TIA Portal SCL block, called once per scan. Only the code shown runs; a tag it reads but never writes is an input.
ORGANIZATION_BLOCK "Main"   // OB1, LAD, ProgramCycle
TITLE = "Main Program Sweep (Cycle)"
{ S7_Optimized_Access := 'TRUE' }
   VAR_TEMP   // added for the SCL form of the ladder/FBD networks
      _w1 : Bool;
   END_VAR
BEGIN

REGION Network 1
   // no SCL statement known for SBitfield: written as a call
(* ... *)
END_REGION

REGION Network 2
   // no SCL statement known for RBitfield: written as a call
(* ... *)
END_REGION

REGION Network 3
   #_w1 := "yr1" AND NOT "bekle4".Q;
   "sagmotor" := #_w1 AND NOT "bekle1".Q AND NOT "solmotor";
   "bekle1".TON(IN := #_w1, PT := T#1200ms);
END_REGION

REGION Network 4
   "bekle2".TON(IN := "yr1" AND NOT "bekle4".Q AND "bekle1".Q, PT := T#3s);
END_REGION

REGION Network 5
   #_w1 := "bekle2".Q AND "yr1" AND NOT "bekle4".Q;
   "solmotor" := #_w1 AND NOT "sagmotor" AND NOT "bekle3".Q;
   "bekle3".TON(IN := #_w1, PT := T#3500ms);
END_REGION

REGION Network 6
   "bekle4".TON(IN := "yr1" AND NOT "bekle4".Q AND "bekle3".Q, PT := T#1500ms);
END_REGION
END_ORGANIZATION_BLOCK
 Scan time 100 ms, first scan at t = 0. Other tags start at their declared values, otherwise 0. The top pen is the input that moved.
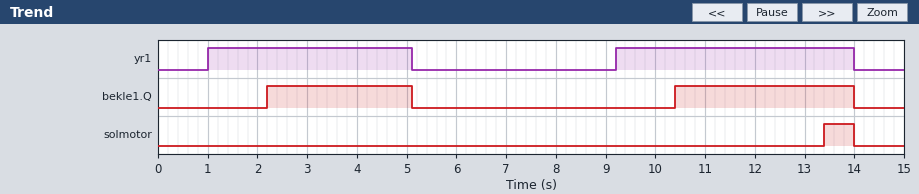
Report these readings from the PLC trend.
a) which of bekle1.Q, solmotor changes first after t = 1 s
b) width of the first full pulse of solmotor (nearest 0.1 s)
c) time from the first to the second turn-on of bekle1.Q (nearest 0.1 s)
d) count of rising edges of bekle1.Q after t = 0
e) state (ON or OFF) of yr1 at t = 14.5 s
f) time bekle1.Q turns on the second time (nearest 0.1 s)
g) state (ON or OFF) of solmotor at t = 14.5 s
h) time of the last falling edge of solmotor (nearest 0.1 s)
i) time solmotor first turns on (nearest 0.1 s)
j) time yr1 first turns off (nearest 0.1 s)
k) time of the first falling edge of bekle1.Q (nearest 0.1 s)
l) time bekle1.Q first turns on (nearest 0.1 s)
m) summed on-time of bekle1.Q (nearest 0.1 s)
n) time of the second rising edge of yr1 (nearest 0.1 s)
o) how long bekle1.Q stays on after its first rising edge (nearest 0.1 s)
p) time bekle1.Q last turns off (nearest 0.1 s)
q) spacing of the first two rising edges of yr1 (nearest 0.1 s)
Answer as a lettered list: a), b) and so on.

a) bekle1.Q
b) 0.6 s
c) 8.2 s
d) 2
e) OFF
f) 10.4 s
g) OFF
h) 14.0 s
i) 13.4 s
j) 5.1 s
k) 5.1 s
l) 2.2 s
m) 6.5 s
n) 9.2 s
o) 2.9 s
p) 14.0 s
q) 8.2 s
